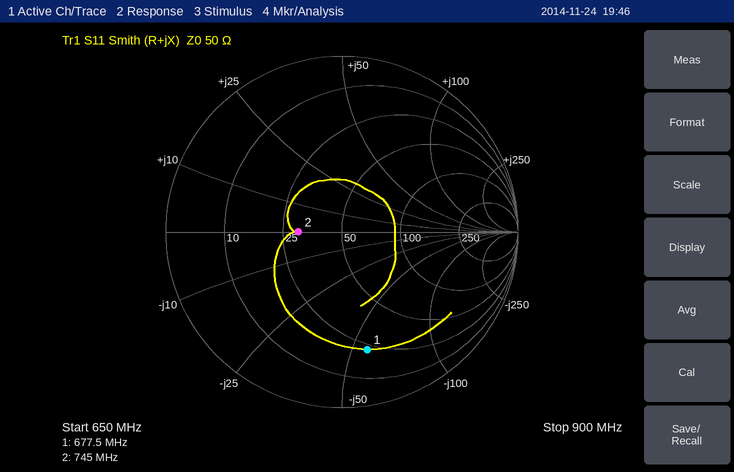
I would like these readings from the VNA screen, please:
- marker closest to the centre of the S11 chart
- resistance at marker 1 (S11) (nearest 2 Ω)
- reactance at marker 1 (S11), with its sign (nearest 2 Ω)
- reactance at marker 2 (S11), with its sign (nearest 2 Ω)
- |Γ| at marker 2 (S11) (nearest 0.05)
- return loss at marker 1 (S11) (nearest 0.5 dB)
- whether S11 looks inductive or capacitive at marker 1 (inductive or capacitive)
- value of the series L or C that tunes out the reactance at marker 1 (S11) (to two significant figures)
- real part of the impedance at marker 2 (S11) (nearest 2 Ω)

marker 2
22 Ω
-56 Ω
0 Ω
0.25
3.5 dB
capacitive
13 nH
30 Ω
